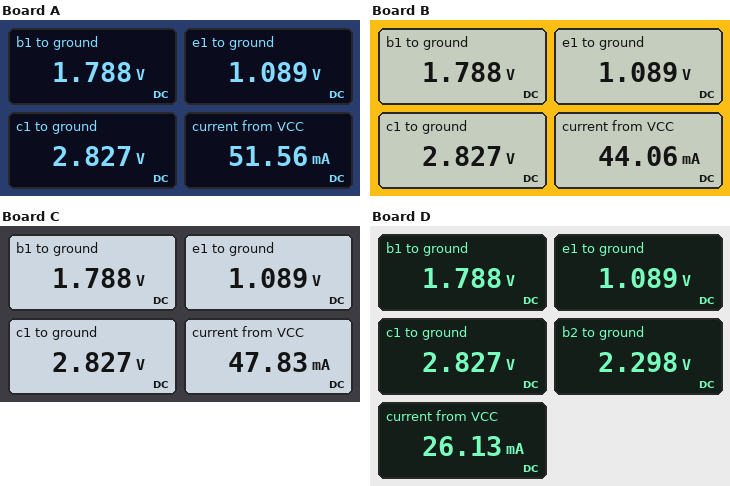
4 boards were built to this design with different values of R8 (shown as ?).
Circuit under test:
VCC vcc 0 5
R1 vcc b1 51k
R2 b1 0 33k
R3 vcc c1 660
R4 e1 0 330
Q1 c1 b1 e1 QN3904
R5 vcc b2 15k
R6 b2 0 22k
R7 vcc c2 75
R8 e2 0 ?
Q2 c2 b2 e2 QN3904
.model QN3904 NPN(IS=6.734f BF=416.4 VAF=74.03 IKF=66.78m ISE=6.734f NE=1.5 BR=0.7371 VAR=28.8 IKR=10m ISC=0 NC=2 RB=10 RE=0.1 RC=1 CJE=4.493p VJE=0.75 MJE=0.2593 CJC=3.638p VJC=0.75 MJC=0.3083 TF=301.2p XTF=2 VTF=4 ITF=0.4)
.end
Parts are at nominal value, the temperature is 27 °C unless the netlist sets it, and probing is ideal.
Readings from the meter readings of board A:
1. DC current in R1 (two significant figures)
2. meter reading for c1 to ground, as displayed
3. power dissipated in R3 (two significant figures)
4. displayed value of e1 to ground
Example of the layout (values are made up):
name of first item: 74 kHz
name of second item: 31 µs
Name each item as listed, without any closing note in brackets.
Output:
DC current in R1: 63 µA
meter reading for c1 to ground, as displayed: 2.827 V
power dissipated in R3: 7.2 mW
displayed value of e1 to ground: 1.089 V
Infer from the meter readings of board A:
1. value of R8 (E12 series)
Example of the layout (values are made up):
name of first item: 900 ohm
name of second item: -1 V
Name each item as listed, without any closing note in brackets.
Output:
value of R8: 6.8 Ω
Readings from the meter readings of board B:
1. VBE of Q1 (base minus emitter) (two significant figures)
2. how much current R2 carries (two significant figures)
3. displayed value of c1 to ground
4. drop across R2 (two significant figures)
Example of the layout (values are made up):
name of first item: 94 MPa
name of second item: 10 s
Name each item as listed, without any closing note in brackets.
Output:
VBE of Q1 (base minus emitter): 700 mV
how much current R2 carries: 54 µA
displayed value of c1 to ground: 2.827 V
drop across R2: 1.8 V
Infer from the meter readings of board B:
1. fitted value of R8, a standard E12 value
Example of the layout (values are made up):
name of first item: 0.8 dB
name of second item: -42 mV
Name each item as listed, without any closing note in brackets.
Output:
fitted value of R8, a standard E12 value: 18 Ω
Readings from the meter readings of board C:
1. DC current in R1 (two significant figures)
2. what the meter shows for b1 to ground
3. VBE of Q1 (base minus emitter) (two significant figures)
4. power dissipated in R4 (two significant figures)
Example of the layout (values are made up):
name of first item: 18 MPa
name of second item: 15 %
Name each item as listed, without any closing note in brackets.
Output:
DC current in R1: 63 µA
what the meter shows for b1 to ground: 1.788 V
VBE of Q1 (base minus emitter): 700 mV
power dissipated in R4: 3.6 mW
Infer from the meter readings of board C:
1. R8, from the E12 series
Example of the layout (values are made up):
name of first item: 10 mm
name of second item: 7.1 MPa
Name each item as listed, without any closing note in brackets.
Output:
R8, from the E12 series: 12 Ω
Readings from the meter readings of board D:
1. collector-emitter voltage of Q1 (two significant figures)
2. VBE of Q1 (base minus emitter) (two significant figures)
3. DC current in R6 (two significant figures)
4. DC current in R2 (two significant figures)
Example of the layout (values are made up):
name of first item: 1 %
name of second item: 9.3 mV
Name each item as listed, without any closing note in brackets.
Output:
collector-emitter voltage of Q1: 1.7 V
VBE of Q1 (base minus emitter): 700 mV
DC current in R6: 100 µA
DC current in R2: 54 µA
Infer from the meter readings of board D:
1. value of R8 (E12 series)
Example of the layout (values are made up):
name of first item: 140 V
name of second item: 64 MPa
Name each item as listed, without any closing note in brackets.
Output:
value of R8: 68 Ω
